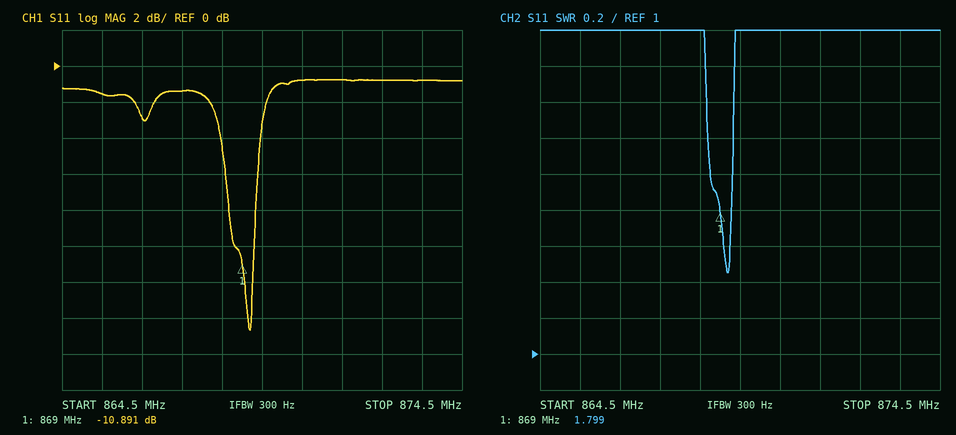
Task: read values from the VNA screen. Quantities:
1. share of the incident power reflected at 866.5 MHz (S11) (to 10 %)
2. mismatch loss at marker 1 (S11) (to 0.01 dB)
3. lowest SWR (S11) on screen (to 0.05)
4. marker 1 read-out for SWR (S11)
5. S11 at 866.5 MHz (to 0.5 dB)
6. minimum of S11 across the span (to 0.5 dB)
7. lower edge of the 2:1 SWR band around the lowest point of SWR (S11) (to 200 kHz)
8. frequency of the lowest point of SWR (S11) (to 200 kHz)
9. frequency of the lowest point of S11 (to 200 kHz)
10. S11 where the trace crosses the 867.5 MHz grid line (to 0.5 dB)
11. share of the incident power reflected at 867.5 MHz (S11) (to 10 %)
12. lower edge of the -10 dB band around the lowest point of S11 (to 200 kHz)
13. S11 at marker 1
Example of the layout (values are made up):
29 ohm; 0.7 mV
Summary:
50 %; 0.37 dB; 1.45; 1.799; -3.0 dB; -14.5 dB; 868.8 MHz; 869.2 MHz; 869.2 MHz; -1.5 dB; 70 %; 868.8 MHz; -10.891 dB
